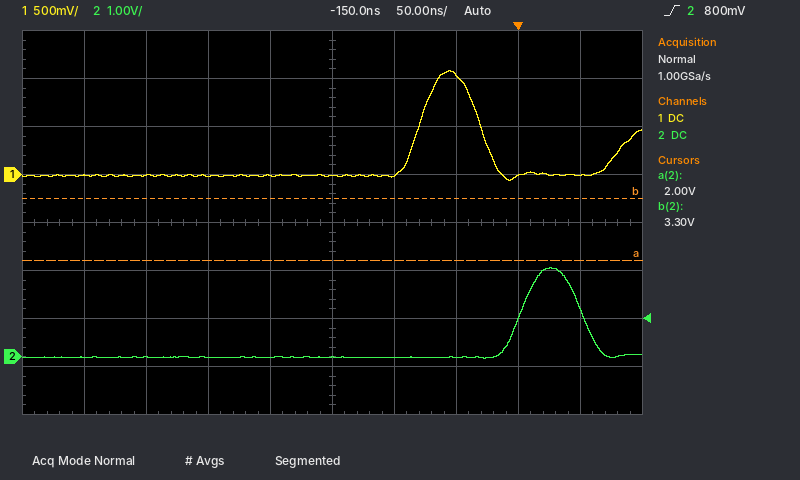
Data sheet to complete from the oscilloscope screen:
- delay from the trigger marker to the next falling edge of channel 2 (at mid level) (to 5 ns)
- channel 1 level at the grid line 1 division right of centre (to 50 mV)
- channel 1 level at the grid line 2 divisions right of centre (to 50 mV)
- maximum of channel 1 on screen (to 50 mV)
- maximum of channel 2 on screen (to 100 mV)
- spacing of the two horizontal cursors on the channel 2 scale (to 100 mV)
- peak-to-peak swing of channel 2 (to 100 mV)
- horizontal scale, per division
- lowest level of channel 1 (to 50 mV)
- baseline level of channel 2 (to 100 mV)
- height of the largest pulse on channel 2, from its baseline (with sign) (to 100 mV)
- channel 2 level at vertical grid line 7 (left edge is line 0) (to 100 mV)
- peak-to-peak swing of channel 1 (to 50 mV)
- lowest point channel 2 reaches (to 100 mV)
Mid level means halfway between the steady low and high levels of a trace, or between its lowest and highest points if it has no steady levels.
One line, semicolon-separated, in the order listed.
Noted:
50 ns; 0 mV; 1.05 V; 1.10 V; 1.9 V; 1.3 V; 1.9 V; 50 ns; -50 mV; 0.0 V; +1.9 V; 0.0 V; 1.15 V; 0.0 V
